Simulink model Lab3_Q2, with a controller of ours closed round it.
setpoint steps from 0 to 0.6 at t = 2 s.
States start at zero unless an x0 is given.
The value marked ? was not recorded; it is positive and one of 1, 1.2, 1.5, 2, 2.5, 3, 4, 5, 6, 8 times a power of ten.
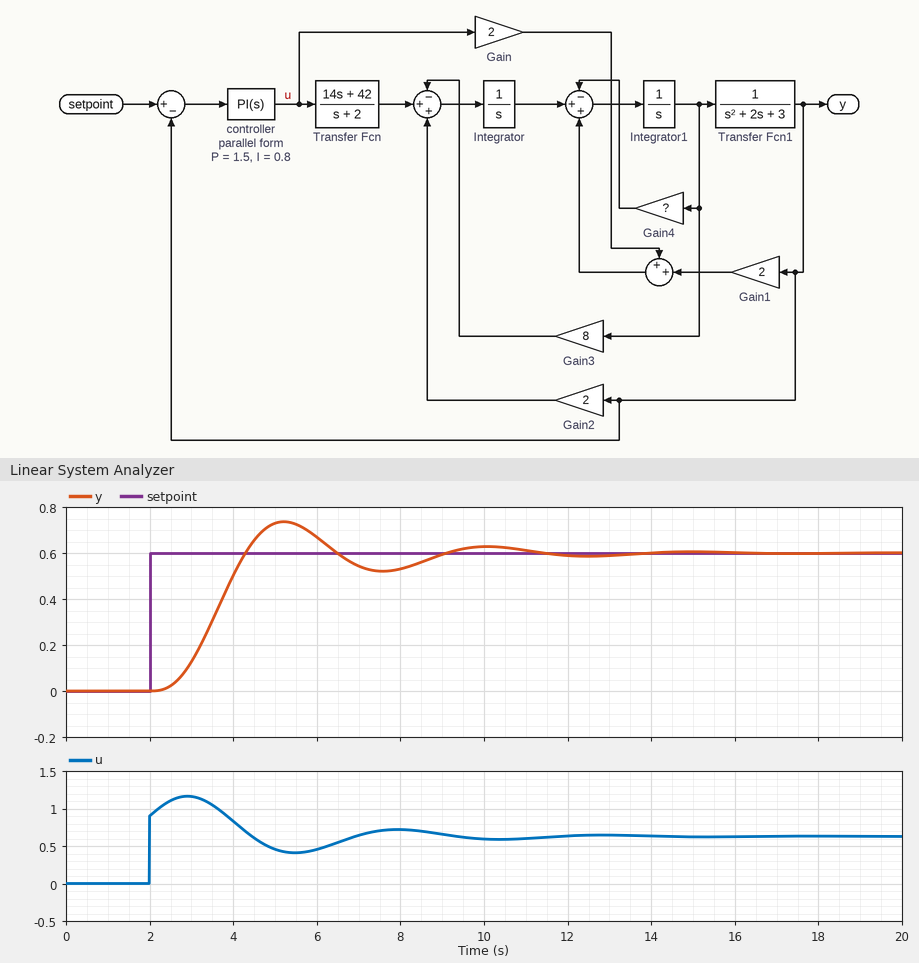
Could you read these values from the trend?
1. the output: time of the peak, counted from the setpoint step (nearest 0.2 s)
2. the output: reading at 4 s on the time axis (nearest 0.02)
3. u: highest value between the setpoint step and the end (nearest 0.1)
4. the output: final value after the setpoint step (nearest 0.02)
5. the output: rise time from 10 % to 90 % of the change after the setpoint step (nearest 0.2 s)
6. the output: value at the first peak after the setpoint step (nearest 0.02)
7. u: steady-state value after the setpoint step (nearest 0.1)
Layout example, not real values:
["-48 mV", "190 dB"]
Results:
["3.2 s", "0.50", "1.2", "0.60", "1.4 s", "0.74", "0.6"]
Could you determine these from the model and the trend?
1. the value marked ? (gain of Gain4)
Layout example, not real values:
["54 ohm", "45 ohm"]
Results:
["12"]
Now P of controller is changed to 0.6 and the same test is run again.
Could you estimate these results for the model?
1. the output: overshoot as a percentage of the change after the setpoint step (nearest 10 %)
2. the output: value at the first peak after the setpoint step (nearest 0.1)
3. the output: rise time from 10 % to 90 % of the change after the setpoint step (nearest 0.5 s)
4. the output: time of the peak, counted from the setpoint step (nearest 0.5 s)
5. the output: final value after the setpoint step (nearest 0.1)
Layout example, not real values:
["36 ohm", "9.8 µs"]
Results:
["30 %", "0.8", "2.0 s", "4.5 s", "0.6"]
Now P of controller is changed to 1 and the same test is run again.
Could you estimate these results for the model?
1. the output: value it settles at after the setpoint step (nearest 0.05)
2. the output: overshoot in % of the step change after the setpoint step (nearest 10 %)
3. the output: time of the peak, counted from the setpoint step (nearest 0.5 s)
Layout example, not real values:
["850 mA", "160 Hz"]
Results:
["0.60", "20 %", "4.0 s"]
